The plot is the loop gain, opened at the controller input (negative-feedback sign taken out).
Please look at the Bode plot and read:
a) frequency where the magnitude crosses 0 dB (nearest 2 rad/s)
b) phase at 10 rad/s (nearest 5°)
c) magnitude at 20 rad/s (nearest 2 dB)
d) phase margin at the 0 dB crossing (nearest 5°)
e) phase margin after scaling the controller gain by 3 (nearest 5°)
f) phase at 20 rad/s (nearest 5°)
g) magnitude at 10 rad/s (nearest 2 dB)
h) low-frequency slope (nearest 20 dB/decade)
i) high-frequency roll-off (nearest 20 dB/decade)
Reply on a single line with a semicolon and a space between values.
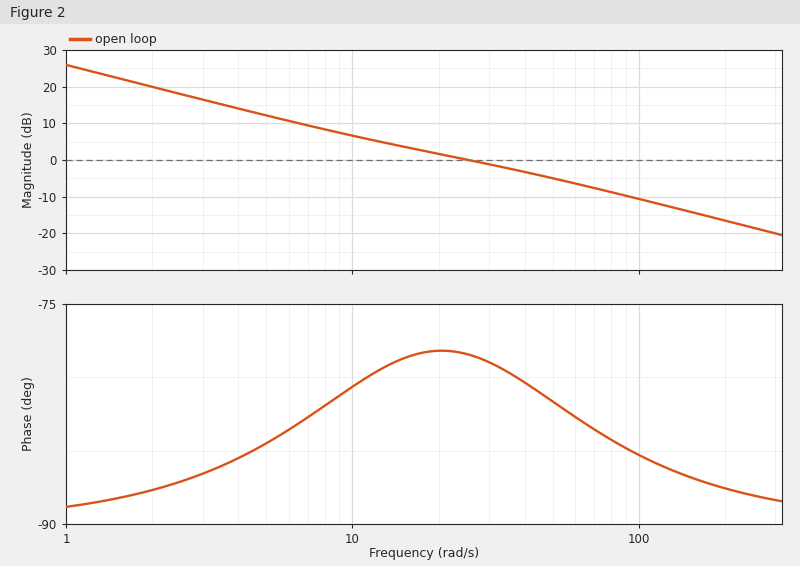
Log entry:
26 rad/s; -80°; 2 dB; 100°; 95°; -80°; 6 dB; -20 dB/decade; -20 dB/decade
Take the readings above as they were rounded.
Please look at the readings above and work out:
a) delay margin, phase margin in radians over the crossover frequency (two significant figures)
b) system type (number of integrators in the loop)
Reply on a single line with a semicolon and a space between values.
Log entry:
0.067 s; 1
